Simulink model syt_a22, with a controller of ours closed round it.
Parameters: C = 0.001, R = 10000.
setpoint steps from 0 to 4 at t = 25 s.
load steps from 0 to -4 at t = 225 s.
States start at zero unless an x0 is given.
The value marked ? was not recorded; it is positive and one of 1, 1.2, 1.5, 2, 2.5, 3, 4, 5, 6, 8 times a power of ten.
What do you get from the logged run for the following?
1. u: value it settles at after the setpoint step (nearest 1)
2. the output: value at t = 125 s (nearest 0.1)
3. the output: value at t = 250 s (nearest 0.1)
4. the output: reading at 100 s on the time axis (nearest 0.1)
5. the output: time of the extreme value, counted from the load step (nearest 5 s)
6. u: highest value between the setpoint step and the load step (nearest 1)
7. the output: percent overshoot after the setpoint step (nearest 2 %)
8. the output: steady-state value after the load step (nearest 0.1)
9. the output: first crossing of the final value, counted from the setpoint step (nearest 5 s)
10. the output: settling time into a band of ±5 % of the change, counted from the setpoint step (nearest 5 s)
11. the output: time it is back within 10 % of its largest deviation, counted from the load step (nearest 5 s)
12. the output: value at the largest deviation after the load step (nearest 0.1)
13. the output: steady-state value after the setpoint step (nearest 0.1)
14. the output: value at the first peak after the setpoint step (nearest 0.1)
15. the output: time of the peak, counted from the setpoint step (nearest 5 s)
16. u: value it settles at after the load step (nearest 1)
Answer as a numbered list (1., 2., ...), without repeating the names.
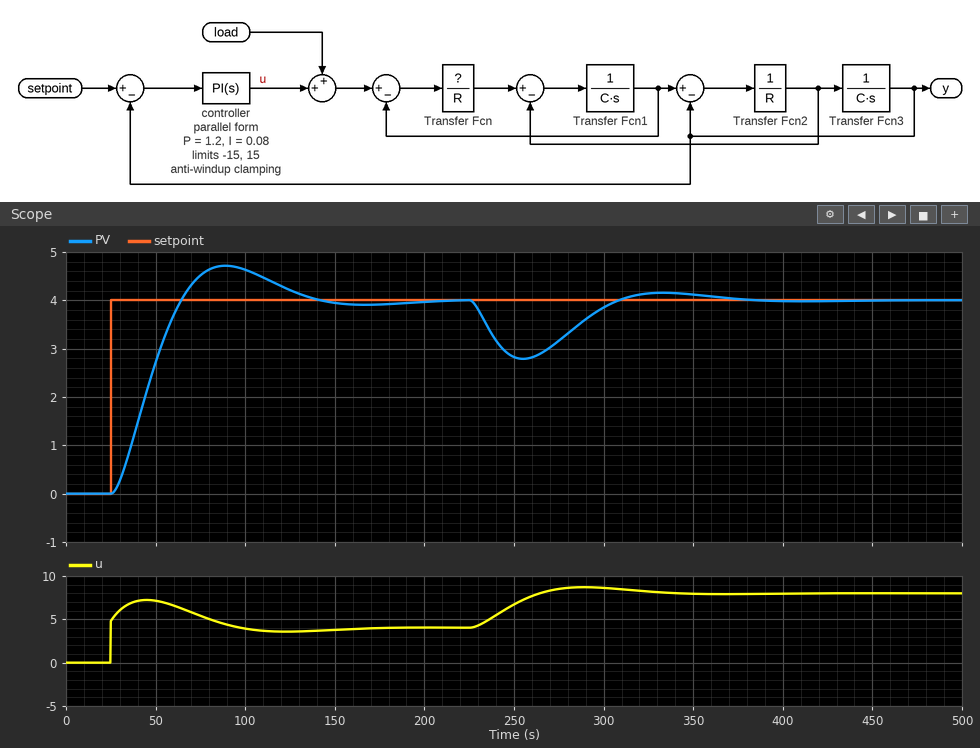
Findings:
1. 4
2. 4.2
3. 2.8
4. 4.6
5. 30 s
6. 7
7. 18 %
8. 4.0
9. 40 s
10. 100 s
11. 125 s
12. 2.8
13. 4.0
14. 4.7
15. 65 s
16. 8
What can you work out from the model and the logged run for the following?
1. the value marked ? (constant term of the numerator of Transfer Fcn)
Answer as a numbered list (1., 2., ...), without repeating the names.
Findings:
1. 0.6
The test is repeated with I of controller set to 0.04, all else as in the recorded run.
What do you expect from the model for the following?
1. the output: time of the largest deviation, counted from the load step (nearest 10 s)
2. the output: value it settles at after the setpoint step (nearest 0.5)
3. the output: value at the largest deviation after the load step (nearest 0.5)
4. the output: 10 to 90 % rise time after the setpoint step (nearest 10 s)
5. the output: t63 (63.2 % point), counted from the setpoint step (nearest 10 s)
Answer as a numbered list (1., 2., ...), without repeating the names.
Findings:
1. 40 s
2. 4.0
3. 2.5
4. 50 s
5. 30 s
